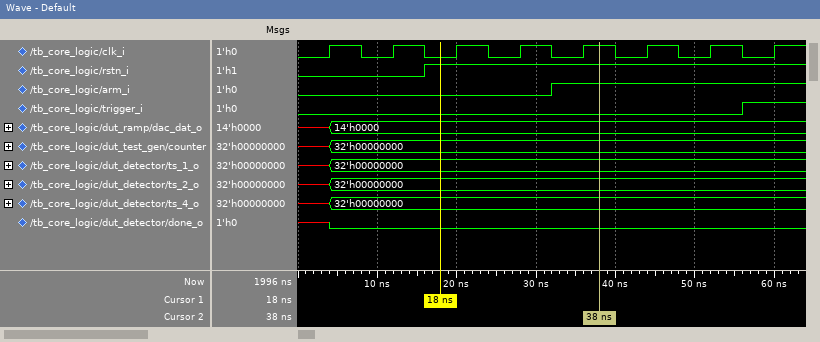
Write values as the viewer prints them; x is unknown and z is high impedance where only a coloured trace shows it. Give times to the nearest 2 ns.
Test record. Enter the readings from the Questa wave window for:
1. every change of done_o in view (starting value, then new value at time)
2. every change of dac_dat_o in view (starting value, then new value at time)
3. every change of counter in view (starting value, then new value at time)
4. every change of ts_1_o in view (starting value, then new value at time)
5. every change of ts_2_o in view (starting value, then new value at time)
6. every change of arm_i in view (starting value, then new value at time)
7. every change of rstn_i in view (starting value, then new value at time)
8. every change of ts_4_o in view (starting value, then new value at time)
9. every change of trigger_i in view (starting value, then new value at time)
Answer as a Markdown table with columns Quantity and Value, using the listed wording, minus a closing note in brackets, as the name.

| Quantity | Value |
|---|---|
| every change of done_o in view | x, 0 at 4 ns |
| every change of dac_dat_o in view | x, 14'h0000 at 4 ns |
| every change of counter in view | x, 32'h00000000 at 4 ns |
| every change of ts_1_o in view | x, 32'h00000000 at 4 ns |
| every change of ts_2_o in view | x, 32'h00000000 at 4 ns |
| every change of arm_i in view | 0, 1 at 32 ns |
| every change of rstn_i in view | 0, 1 at 16 ns |
| every change of ts_4_o in view | x, 32'h00000000 at 4 ns |
| every change of trigger_i in view | 0, 1 at 56 ns |
